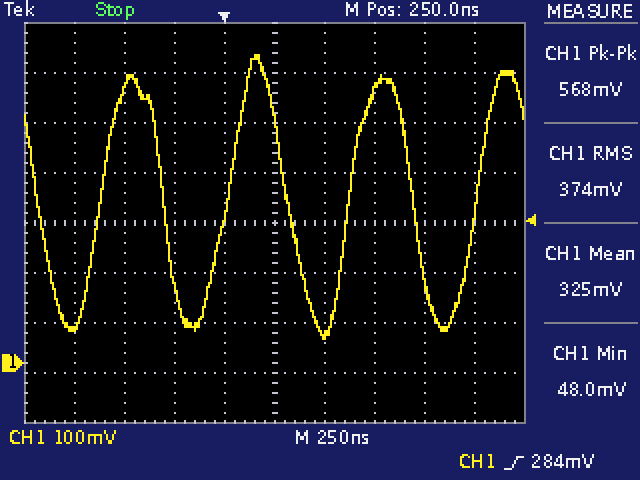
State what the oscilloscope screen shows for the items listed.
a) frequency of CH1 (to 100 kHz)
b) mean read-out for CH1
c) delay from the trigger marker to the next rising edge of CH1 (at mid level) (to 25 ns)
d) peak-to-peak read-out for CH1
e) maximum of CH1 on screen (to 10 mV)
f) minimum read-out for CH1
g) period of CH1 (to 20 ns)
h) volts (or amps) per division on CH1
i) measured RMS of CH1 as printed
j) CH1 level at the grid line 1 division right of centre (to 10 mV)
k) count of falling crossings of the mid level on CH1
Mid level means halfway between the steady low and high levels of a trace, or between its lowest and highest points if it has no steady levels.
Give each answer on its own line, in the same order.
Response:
1.6 MHz
325 mV
25 ns
568 mV
620 mV
48.0 mV
620 ns
100 mV
374 mV
60 mV
4
